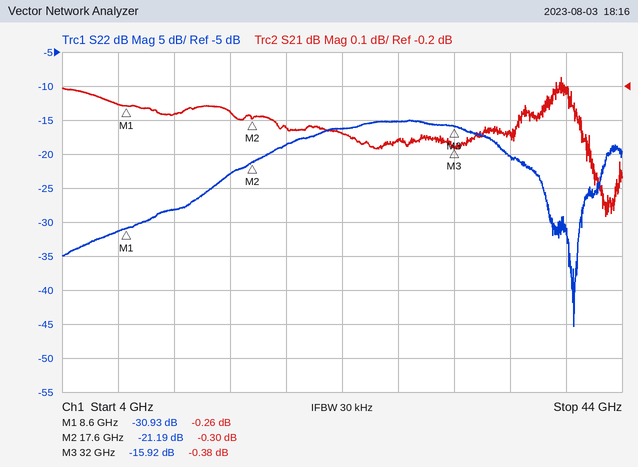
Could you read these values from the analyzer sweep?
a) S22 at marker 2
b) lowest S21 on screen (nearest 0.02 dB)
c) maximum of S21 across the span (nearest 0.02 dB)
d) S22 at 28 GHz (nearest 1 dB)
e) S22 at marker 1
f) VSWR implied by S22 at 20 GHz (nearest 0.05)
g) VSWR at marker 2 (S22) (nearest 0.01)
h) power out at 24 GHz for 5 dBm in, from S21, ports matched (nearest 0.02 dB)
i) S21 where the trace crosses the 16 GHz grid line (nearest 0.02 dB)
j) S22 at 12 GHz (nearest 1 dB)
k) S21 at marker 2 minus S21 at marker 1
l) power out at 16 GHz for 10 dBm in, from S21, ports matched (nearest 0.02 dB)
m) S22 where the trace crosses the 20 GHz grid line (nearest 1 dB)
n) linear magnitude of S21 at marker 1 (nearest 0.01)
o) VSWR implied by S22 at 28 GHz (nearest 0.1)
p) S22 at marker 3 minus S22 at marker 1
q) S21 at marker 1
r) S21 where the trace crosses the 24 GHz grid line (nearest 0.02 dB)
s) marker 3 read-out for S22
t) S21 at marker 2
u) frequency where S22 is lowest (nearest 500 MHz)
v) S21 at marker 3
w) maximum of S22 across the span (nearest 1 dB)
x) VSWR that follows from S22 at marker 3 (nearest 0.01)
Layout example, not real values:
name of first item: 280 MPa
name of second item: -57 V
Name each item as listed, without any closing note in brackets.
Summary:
S22 at marker 2: -21.19 dB
lowest S21 on screen: -0.58 dB
maximum of S21 across the span: -0.18 dB
S22 at 28 GHz: -15 dB
S22 at marker 1: -30.93 dB
VSWR implied by S22 at 20 GHz: 1.25
VSWR at marker 2 (S22): 1.19
power out at 24 GHz for 5 dBm in, from S21, ports matched: 4.66 dBm
S21 where the trace crosses the 16 GHz grid line: -0.28 dB
S22 at 12 GHz: -28 dB
S21 at marker 2 minus S21 at marker 1: -0.04 dB
power out at 16 GHz for 10 dBm in, from S21, ports matched: 9.72 dBm
S22 where the trace crosses the 20 GHz grid line: -19 dB
linear magnitude of S21 at marker 1: 0.97
VSWR implied by S22 at 28 GHz: 1.4
S22 at marker 3 minus S22 at marker 1: 15.01 dB
S21 at marker 1: -0.26 dB
S21 where the trace crosses the 24 GHz grid line: -0.34 dB
marker 3 read-out for S22: -15.92 dB
S21 at marker 2: -0.30 dB
frequency where S22 is lowest: 40.5 GHz
S21 at marker 3: -0.38 dB
maximum of S22 across the span: -15 dB
VSWR that follows from S22 at marker 3: 1.38
